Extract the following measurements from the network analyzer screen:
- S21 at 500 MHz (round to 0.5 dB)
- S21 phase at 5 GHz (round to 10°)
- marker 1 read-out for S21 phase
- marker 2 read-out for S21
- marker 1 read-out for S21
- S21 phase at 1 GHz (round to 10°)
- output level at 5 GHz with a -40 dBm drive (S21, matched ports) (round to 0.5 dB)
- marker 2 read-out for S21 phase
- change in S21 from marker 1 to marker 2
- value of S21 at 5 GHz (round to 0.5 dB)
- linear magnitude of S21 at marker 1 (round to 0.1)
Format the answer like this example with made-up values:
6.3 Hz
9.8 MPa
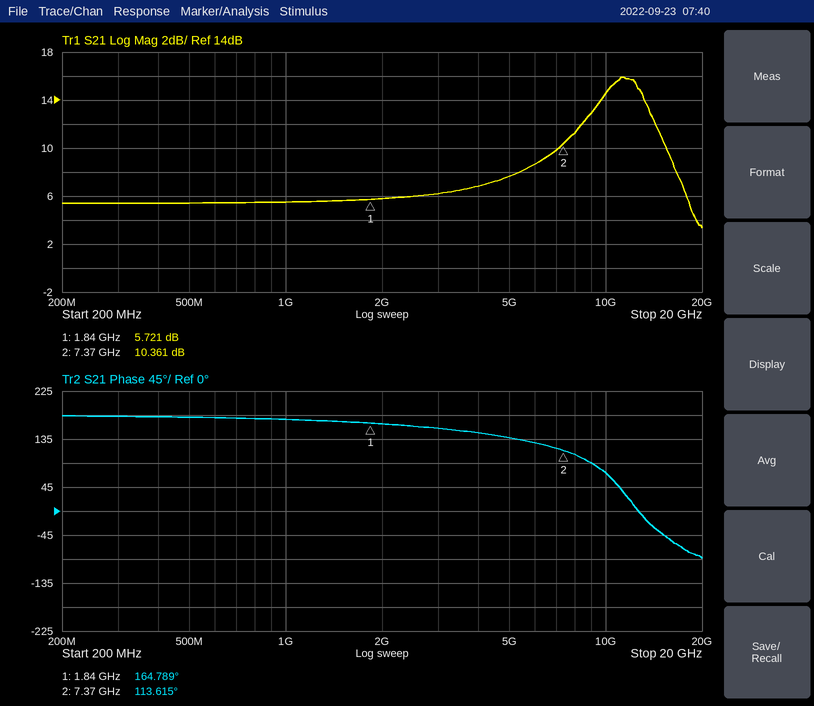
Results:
5.5 dB
140°
164.789°
10.361 dB
5.721 dB
170°
-32.5 dBm
113.615°
4.640 dB
7.5 dB
1.9
